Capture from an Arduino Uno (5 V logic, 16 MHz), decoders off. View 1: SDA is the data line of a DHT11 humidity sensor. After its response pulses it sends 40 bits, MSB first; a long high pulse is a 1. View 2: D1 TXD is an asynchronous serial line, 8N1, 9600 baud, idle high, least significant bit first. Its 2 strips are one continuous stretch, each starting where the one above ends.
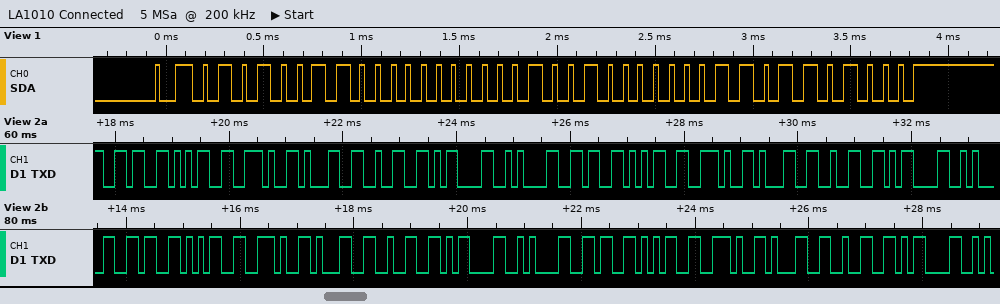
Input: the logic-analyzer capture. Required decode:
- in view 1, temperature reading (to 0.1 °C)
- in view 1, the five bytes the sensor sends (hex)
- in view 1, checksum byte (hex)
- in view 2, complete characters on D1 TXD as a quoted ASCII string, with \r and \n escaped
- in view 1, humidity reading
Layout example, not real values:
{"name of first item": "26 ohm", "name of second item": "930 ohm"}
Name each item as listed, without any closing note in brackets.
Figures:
{"in view 1, temperature reading": "18.3 °C", "in view 1, the five bytes the sensor sends": "53 00 12 03 68", "in view 1, checksum byte": "0x68", "in view 2, complete characters on D1 TXD as a quoted ASCII string, with \\r and \\n escaped": "\"65.12\\r\\n65.12\\r\\n65.12\\r\\n65.12\\r\"", "in view 1, humidity reading": "83 %"}
